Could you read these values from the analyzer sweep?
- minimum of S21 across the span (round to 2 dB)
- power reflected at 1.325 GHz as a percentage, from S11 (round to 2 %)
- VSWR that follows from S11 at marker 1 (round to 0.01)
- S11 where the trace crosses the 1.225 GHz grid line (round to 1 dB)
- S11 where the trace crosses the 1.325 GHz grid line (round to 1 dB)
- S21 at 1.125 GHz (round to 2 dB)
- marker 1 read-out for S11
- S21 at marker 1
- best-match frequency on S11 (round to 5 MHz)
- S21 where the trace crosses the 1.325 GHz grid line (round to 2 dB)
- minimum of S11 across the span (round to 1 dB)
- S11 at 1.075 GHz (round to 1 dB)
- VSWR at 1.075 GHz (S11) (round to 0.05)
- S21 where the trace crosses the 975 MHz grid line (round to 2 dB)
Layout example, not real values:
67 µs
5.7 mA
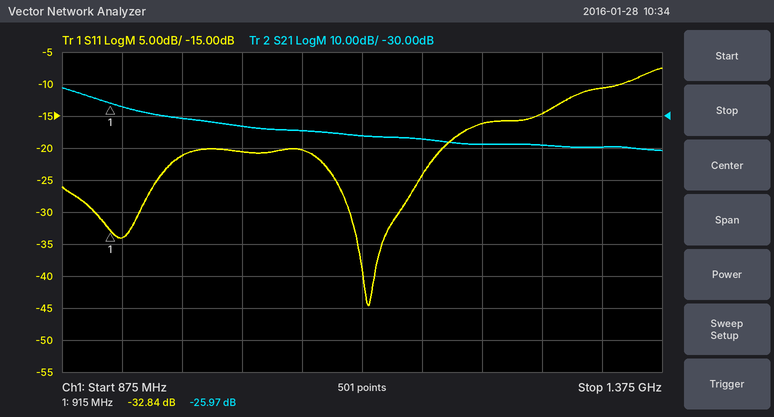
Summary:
-40 dB
8 %
1.05
-16 dB
-11 dB
-36 dB
-32.84 dB
-25.97 dB
1.130 GHz
-40 dB
-45 dB
-20 dB
1.20
-30 dB
